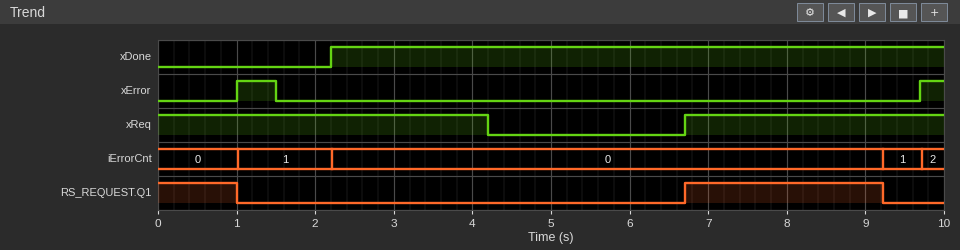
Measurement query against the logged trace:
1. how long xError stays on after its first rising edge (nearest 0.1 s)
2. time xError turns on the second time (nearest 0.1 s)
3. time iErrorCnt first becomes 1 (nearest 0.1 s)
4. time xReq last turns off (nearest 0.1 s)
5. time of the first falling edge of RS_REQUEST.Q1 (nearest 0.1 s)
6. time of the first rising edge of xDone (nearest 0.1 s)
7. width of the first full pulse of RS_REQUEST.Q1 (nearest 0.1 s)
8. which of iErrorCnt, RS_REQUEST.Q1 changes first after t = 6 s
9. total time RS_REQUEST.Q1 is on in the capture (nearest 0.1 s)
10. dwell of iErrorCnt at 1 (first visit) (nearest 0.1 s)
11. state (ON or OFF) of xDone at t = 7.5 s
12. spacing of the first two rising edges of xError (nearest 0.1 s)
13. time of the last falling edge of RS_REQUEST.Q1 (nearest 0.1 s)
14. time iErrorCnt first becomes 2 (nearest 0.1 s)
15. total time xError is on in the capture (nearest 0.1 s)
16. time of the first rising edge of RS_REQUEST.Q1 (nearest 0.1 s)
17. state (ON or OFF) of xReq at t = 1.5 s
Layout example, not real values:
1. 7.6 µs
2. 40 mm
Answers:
1. 0.5 s
2. 9.7 s
3. 1.0 s
4. 4.2 s
5. 1.0 s
6. 2.2 s
7. 2.5 s
8. RS_REQUEST.Q1
9. 3.5 s
10. 1.2 s
11. ON
12. 8.7 s
13. 9.2 s
14. 9.7 s
15. 0.8 s
16. 6.7 s
17. ON
